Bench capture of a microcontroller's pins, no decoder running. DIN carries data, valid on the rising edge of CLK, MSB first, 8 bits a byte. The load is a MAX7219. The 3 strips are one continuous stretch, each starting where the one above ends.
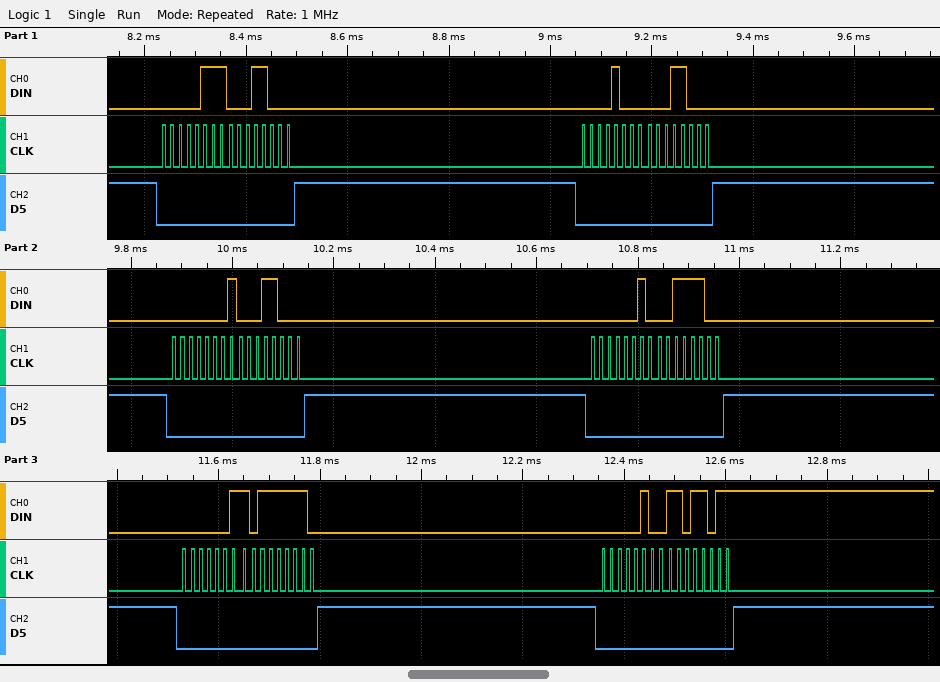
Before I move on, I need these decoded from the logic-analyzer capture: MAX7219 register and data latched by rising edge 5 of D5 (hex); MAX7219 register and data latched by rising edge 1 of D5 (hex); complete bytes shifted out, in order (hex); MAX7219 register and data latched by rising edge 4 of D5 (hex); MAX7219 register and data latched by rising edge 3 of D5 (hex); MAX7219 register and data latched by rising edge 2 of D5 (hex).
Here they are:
register 0x3, data 0x7E
register 0x7, data 0x18
07 18 08 18 01 18 02 3C 03 7E 04 DB
register 0x2, data 0x3C
register 0x1, data 0x18
register 0x8, data 0x18
